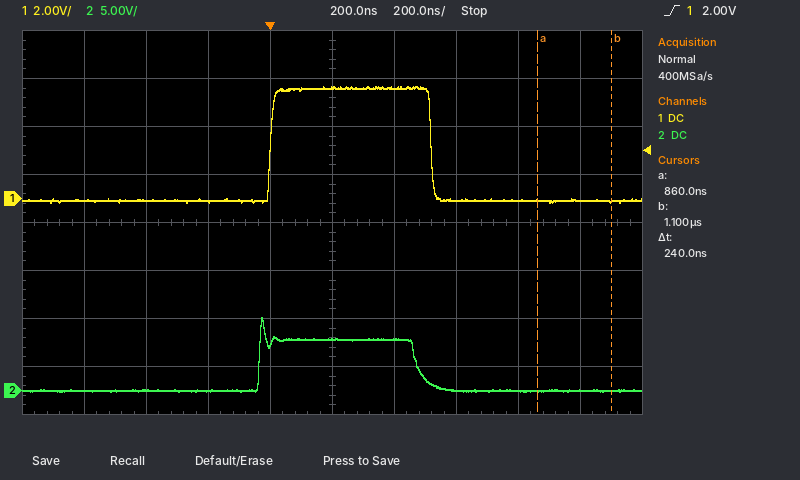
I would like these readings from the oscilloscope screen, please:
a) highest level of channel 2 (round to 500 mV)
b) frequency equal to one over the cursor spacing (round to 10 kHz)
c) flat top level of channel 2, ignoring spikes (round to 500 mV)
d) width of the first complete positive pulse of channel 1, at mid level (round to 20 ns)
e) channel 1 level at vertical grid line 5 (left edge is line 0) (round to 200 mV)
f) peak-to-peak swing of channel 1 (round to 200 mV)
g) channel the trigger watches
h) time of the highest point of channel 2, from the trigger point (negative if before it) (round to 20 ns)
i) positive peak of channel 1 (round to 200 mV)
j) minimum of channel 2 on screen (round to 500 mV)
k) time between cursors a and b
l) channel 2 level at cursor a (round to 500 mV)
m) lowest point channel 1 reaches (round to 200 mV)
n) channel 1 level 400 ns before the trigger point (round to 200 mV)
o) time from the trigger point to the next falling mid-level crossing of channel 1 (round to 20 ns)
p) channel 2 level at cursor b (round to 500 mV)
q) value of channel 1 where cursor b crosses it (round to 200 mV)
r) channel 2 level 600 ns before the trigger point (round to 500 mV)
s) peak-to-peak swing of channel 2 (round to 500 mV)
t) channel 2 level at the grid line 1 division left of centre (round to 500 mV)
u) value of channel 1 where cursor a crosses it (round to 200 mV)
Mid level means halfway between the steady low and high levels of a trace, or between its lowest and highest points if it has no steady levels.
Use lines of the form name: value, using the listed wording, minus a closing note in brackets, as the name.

highest level of channel 2: 7.5 V
frequency equal to one over the cursor spacing: 4.17 MHz
flat top level of channel 2, ignoring spikes: 5.5 V
width of the first complete positive pulse of channel 1, at mid level: 520 ns
channel 1 level at vertical grid line 5 (left edge is line 0): 4.6 V
peak-to-peak swing of channel 1: 4.8 V
channel the trigger watches: channel 1
time of the highest point of channel 2, from the trigger point (negative if before it): -20 ns
positive peak of channel 1: 4.6 V
minimum of channel 2 on screen: 0.0 V
time between cursors a and b: 240 ns
channel 2 level at cursor a: 0.0 V
lowest point channel 1 reaches: -200 mV
channel 1 level 400 ns before the trigger point: 0.0 V
time from the trigger point to the next falling mid-level crossing of channel 1: 520 ns
channel 2 level at cursor b: 0.0 V
value of channel 1 where cursor b crosses it: -200 mV
channel 2 level 600 ns before the trigger point: 0.0 V
peak-to-peak swing of channel 2: 7.5 V
channel 2 level at the grid line 1 division left of centre: 5.0 V
value of channel 1 where cursor a crosses it: 0.0 V
